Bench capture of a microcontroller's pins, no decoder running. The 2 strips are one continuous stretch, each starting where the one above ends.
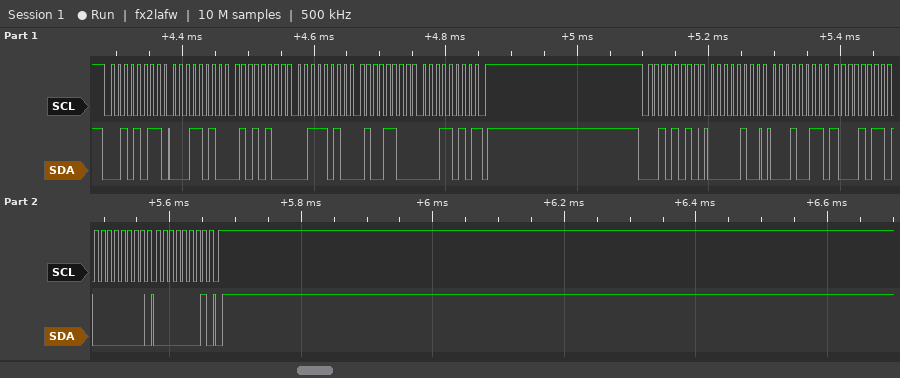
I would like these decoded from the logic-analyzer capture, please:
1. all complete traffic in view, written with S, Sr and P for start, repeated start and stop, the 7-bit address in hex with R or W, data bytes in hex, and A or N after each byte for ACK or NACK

S 15R A 1A A 54 A 3A A 4C A 1A N P S 15W A 04 A 13 A 8B A 00 A 01 A P
